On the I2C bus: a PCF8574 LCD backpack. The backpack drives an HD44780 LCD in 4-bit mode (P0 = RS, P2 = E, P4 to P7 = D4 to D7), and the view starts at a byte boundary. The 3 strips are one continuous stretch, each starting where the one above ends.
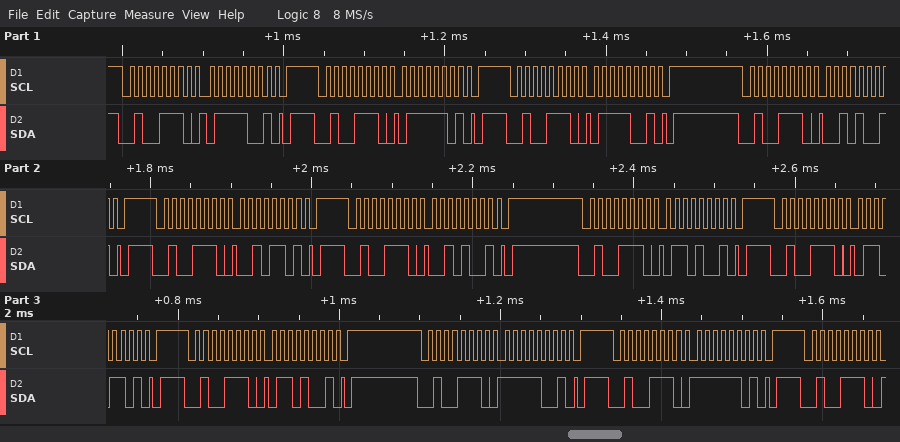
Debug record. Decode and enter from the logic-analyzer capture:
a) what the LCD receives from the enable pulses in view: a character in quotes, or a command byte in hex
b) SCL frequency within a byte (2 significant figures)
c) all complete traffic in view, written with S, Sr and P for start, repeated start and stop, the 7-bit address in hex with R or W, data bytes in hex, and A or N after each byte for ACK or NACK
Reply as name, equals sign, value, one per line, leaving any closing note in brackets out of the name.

what the LCD receives from the enable pulses in view: a character in quotes, or a command byte in hex = 'r'
SCL frequency within a byte = 100 kHz
all complete traffic in view, written with S, Sr and P for start, repeated start and stop, the 7-bit address in hex with R or W, data bytes in hex, and A or N after each byte for ACK or NACK = S 27W A 79 A P S 27W A 7D A P S 27W A 79 A P S 27W A 29 A P S 27W A 2D A P S 27W A 29 A P S 27W A 69 A P S 27W A 6D A P S 27W A 69 A P S 27W A F9 A P S 27W A FD A P S 27W A
